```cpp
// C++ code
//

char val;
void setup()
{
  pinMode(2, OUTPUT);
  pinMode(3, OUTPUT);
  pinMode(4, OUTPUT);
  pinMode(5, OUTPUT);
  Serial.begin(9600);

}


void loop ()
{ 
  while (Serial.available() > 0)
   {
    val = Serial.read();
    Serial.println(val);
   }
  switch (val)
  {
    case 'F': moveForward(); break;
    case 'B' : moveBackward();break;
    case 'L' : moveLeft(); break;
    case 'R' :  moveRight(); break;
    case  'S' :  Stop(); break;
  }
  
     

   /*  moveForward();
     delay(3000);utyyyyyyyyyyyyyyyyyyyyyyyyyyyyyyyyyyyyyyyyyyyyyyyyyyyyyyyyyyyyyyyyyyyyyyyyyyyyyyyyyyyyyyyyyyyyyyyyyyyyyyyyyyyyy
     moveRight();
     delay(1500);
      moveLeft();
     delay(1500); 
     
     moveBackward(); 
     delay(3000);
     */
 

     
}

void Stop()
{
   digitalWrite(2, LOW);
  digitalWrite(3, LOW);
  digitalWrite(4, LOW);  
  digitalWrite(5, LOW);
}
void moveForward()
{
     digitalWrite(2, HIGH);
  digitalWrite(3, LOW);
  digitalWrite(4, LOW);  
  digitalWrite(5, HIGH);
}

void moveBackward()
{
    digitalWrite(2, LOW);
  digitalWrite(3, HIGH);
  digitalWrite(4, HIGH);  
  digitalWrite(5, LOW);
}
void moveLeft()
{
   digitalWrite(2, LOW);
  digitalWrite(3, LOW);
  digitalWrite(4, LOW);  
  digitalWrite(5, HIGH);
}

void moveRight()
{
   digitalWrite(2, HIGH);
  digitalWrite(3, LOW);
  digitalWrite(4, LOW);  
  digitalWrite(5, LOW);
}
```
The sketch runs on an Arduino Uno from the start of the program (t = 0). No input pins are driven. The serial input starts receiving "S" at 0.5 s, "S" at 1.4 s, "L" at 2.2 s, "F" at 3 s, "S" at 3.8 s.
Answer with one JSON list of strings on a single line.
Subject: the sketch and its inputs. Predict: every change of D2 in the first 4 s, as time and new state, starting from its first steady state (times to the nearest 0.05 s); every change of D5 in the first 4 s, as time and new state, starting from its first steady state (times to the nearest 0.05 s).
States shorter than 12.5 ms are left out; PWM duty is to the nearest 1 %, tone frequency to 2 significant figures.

["0 s low; 3 s high; 3.8 s low", "0 s low; 2.2 s high; 3.8 s low"]
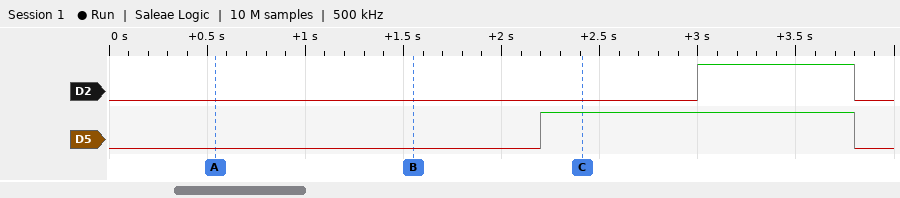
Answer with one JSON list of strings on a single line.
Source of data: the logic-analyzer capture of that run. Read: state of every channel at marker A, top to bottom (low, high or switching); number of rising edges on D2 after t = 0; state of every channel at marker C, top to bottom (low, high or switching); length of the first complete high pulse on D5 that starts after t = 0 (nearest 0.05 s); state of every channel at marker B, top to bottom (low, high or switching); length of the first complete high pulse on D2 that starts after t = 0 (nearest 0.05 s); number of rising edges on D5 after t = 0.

["D2 low, D5 low", "1", "D2 low, D5 high", "1.60 s", "D2 low, D5 low", "0.80 s", "1"]
